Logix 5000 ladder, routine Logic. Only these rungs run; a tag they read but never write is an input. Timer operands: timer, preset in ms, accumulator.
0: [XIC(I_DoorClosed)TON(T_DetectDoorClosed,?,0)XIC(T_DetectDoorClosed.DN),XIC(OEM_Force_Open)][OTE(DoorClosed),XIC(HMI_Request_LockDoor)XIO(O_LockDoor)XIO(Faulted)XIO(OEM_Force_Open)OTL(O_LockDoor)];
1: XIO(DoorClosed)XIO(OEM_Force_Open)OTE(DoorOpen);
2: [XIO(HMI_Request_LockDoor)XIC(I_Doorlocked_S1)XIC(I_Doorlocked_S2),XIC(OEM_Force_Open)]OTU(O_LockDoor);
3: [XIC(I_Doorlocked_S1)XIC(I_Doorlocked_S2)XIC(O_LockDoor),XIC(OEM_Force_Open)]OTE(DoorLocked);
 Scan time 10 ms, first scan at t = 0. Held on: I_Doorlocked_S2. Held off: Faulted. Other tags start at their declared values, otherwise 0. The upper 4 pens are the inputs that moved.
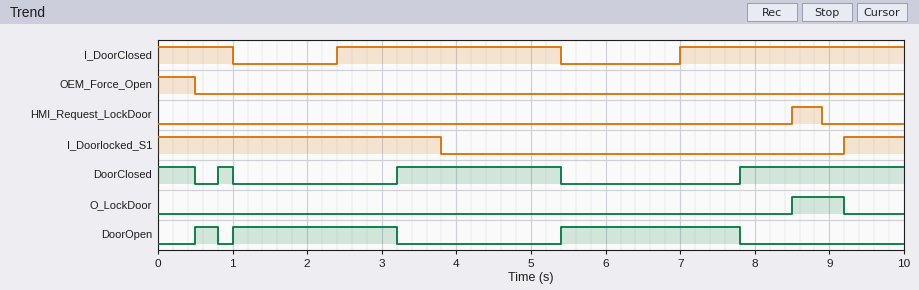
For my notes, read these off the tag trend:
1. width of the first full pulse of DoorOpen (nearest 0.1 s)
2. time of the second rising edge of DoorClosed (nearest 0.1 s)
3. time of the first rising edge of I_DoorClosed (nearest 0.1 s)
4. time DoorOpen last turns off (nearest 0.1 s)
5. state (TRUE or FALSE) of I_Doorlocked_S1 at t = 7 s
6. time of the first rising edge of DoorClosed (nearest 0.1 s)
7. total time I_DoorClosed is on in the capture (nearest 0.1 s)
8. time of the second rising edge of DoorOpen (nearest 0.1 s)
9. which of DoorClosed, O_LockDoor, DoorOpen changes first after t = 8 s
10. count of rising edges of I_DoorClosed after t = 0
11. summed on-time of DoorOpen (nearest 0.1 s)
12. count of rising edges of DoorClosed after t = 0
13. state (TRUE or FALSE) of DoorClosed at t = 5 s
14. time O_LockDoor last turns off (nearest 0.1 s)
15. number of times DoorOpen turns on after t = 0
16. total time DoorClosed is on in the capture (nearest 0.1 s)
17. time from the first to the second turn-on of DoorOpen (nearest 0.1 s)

0.3 s
3.2 s
2.4 s
7.8 s
FALSE
0.8 s
7.0 s
1.0 s
O_LockDoor
2
4.9 s
3
TRUE
9.2 s
3
5.1 s
0.5 s
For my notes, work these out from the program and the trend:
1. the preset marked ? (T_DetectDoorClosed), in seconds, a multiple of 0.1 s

0.8 s
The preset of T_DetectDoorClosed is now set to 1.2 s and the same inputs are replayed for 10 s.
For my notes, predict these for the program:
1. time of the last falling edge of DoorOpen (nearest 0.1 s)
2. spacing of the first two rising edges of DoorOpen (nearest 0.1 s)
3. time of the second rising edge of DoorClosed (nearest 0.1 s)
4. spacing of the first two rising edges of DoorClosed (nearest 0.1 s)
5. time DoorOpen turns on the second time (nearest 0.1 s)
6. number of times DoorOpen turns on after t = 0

8.2 s
4.9 s
8.2 s
4.6 s
5.4 s
2
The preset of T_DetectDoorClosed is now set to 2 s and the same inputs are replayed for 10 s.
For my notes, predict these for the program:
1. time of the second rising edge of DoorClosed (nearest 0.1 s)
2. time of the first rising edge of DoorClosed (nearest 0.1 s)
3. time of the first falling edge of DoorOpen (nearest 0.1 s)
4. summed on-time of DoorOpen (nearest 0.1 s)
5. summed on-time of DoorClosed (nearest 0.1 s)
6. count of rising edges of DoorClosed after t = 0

9.0 s
4.4 s
4.4 s
7.5 s
2.5 s
2
